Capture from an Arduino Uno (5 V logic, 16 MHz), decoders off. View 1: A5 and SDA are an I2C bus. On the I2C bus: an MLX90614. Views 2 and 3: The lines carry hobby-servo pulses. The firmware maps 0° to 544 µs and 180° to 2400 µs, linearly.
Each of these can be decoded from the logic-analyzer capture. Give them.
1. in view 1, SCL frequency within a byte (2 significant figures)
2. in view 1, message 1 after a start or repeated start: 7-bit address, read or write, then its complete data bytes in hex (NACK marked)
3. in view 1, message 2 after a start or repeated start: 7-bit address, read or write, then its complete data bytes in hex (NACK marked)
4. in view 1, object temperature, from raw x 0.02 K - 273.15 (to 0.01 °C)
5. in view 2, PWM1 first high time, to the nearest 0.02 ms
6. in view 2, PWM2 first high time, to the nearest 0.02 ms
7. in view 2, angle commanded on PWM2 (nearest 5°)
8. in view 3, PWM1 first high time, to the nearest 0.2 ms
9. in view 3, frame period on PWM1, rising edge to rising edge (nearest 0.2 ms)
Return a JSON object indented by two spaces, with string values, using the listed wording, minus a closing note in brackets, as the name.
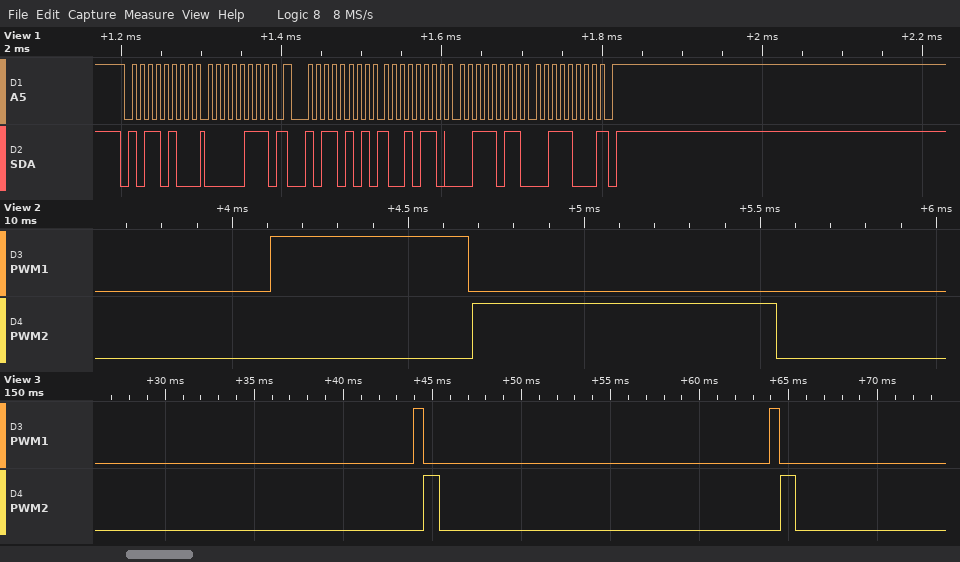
{
  "in view 1, SCL frequency within a byte": "100 kHz",
  "in view 1, message 1 after a start or repeated start: 7-bit address, read or write, then its complete data bytes in hex": "0x5A write: 07",
  "in view 1, message 2 after a start or repeated start: 7-bit address, read or write, then its complete data bytes in hex": "0x5A read: 96 3B 38 NACK",
  "in view 1, object temperature, from raw x 0.02 K - 273.15": "31.93 °C",
  "in view 2, PWM1 first high time, to the nearest 0.02 ms": "0.56 ms",
  "in view 2, PWM2 first high time, to the nearest 0.02 ms": "0.86 ms",
  "in view 2, angle commanded on PWM2": "30°",
  "in view 3, PWM1 first high time, to the nearest 0.2 ms": "0.6 ms",
  "in view 3, frame period on PWM1, rising edge to rising edge": "20.0 ms"
}
